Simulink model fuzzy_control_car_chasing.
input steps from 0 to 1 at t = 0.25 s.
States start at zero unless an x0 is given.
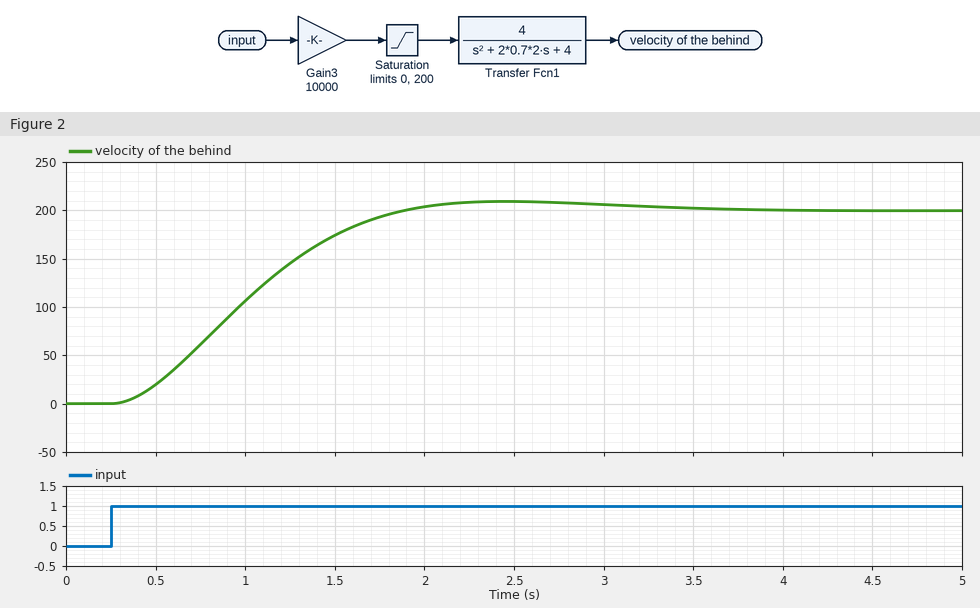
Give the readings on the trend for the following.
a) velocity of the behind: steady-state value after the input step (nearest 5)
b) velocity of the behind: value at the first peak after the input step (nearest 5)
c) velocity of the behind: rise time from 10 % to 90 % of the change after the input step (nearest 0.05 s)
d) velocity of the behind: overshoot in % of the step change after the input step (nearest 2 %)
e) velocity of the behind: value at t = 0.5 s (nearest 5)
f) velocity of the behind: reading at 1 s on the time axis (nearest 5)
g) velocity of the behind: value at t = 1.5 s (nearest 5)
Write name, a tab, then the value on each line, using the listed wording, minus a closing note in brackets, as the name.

velocity of the behind: steady-state value after the input step	200
velocity of the behind: value at the first peak after the input step	210
velocity of the behind: rise time from 10 % to 90 % of the change after the input step	1.05 s
velocity of the behind: overshoot in % of the step change after the input step	4 %
velocity of the behind: value at t = 0.5 s	20
velocity of the behind: reading at 1 s on the time axis	105
velocity of the behind: value at t = 1.5 s	175
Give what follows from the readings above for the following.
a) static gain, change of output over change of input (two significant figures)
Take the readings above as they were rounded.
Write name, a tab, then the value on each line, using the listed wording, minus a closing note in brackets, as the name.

static gain, change of output over change of input	200
